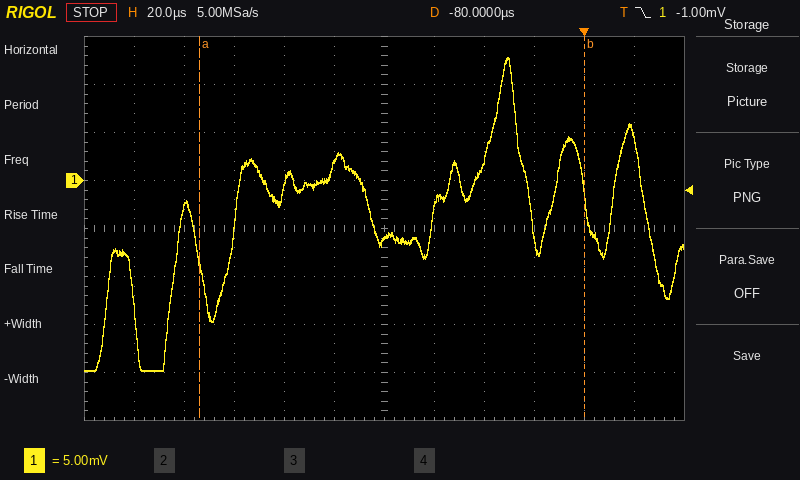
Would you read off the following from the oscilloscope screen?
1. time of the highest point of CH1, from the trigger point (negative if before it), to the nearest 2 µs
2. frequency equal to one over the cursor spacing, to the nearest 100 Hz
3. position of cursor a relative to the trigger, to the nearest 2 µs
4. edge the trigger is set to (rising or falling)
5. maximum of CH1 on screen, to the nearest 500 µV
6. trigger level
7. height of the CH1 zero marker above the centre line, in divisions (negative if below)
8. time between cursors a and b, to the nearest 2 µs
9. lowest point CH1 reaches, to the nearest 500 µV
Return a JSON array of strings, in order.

["-30 µs", "6.5 kHz", "-154 µs", "falling", "13.0 mV", "-1.00 mV", "+1.0 div", "154 µs", "-20.0 mV"]
